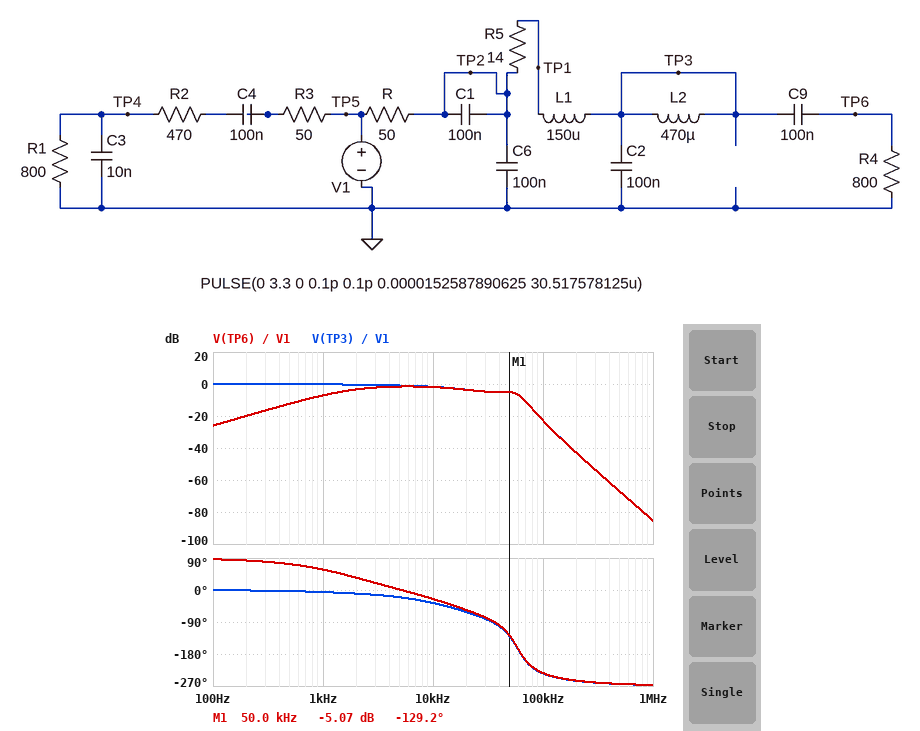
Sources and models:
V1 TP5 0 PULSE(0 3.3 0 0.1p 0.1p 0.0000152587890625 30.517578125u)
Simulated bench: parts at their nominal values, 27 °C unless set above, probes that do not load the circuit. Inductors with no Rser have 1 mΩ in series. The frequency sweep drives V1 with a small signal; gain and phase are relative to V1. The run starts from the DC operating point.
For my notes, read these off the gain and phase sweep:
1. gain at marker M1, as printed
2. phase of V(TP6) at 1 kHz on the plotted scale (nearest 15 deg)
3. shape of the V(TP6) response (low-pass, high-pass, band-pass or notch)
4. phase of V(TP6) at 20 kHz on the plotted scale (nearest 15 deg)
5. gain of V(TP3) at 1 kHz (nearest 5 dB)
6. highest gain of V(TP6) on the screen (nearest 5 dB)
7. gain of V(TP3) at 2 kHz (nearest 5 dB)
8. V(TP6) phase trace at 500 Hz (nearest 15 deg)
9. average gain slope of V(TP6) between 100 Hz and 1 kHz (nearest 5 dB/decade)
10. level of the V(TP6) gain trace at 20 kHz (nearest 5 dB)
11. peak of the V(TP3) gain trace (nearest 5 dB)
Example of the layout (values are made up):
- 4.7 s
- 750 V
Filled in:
- -5.07 dB
- 60 deg
- band-pass
- -60 deg
- 0 dB
- 0 dB
- 0 dB
- 75 deg
- 20 dB/decade
- -5 dB
- 0 dB
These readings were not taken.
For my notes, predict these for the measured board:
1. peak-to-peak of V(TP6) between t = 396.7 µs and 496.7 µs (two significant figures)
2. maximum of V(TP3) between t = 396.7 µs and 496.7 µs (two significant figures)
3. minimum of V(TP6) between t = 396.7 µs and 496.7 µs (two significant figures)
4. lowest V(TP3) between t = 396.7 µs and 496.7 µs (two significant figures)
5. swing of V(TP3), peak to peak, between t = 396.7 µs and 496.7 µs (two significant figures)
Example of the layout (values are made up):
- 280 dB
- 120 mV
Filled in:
- 2.3 V
- 2.8 V
- -1.1 V
- 500 mV
- 2.3 V
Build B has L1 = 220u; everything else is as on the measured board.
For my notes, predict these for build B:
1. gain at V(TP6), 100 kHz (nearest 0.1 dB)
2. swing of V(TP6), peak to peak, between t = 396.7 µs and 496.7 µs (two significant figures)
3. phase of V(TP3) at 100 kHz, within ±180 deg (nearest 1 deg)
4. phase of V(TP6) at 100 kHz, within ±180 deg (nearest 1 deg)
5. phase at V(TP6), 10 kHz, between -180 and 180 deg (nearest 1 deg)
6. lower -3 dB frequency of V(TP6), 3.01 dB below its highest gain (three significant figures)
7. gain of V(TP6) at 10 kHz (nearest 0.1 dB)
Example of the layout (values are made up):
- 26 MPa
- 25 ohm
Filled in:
- -27.1 dB
- 2.8 V
- 119 deg
- 120 deg
- -26 deg
- 1.57 kHz
- -1.7 dB
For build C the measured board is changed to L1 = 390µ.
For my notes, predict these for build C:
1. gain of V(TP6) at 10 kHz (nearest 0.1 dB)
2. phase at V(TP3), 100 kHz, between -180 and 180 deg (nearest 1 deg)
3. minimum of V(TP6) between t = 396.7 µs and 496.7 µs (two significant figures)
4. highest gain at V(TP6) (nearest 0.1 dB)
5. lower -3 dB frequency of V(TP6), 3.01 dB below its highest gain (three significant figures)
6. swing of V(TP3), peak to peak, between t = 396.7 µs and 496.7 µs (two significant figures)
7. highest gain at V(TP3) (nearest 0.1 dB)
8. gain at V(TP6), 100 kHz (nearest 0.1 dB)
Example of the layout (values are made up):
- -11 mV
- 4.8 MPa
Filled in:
- -1.3 dB
- 114 deg
- -1.7 V
- -1.1 dB
- 1.70 kHz
- 3.4 V
- 0 dB
- -33.0 dB
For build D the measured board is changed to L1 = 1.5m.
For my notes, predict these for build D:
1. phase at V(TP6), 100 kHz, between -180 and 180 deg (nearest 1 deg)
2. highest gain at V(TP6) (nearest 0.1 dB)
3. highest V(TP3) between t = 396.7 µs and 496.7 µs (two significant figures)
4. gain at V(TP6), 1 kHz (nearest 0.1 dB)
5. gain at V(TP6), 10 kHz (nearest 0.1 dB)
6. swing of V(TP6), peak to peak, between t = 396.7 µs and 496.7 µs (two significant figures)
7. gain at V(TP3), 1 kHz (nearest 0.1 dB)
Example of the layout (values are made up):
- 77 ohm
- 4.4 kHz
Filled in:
- 111 deg
- 3.2 dB
- 1.9 V
- -7.0 dB
- 2.1 dB
- 590 mV
- -0.1 dB
